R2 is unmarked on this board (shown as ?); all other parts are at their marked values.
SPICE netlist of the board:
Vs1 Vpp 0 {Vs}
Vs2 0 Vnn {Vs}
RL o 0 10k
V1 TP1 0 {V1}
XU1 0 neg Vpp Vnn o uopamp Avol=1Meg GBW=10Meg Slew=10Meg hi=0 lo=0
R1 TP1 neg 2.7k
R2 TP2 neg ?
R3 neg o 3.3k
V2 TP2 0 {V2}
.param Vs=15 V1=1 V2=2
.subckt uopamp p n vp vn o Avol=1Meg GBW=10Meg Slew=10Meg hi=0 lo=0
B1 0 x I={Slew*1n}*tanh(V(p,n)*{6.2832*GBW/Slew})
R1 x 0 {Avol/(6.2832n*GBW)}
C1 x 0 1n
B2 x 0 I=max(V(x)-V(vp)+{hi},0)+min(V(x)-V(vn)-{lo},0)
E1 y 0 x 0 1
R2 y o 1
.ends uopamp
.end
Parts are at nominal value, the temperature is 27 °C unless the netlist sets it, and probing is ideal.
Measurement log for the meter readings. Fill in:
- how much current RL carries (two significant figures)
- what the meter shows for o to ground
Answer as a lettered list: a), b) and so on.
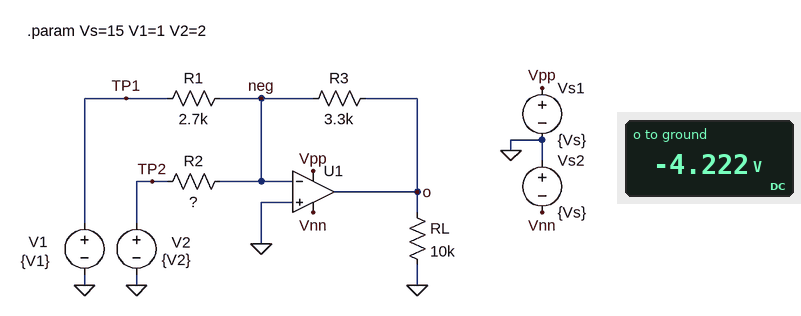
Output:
a) 420 µA
b) -4.222 V
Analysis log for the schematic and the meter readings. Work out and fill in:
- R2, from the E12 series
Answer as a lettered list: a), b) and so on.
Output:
a) 2.2 kΩ
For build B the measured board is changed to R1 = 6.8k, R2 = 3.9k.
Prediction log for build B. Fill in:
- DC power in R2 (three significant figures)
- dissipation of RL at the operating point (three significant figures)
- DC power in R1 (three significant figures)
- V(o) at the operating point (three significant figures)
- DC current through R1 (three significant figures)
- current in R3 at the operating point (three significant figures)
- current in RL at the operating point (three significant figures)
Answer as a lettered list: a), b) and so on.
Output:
a) 1.03 mW
b) 474 µW
c) 147 µW
d) -2.18 V
e) 147 µA
f) 660 µA
g) 218 µA
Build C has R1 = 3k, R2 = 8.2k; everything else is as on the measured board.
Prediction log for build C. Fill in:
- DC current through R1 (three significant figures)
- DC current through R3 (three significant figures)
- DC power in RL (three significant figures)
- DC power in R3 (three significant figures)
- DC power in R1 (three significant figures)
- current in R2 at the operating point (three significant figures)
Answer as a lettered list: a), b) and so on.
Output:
a) 333 µA
b) 577 µA
c) 363 µW
d) 1.10 mW
e) 333 µW
f) 244 µA
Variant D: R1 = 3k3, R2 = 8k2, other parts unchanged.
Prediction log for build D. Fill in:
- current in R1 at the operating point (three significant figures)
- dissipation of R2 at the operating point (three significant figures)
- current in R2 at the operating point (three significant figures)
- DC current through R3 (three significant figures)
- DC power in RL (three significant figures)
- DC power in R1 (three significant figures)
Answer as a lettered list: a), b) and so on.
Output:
a) 303 µA
b) 488 µW
c) 244 µA
d) 547 µA
e) 326 µW
f) 303 µW
